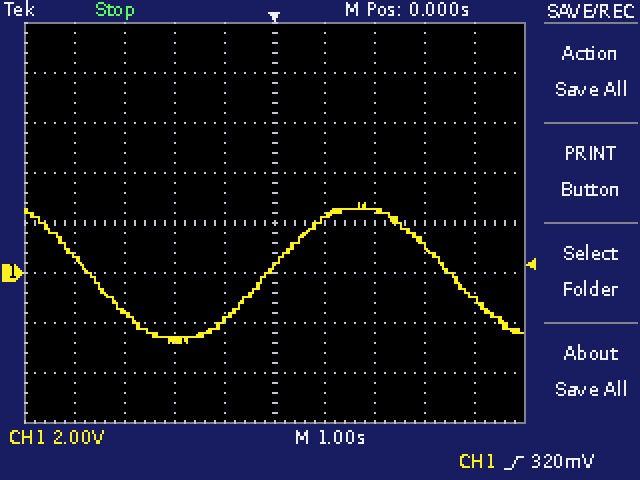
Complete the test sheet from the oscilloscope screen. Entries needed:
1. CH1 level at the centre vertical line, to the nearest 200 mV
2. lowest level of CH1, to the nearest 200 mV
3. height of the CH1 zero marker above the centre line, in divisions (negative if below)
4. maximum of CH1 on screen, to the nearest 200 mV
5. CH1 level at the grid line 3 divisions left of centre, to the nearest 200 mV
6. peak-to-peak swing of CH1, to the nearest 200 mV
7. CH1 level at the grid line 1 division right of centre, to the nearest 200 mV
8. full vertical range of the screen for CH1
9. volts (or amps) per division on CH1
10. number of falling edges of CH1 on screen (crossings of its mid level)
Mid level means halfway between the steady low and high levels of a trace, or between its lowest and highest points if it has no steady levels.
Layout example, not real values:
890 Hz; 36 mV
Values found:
200 mV; -2.8 V; -1.0 div; 2.8 V; -1.6 V; 5.6 V; 2.2 V; 16 V; 2 V; 2
